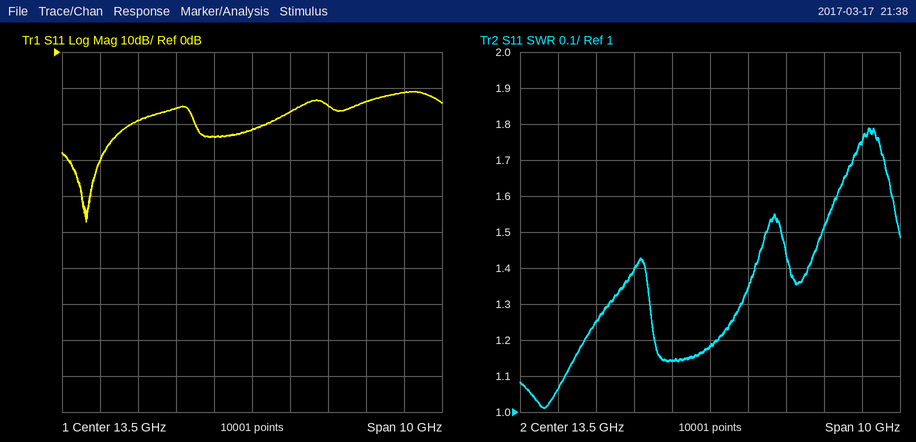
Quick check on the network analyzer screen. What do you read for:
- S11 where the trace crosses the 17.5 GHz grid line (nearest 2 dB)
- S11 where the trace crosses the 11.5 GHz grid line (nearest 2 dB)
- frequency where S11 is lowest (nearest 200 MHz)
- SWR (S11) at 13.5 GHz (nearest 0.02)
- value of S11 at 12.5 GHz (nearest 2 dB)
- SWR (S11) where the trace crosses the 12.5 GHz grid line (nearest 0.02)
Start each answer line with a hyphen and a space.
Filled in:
- -12 dB
- -16 dB
- 9.2 GHz
- 1.18
- -24 dB
- 1.14
